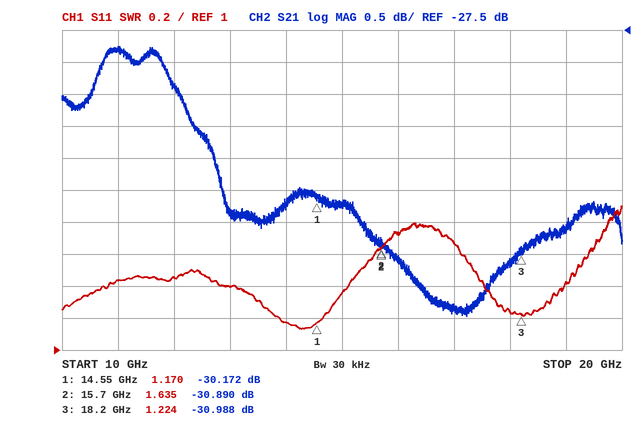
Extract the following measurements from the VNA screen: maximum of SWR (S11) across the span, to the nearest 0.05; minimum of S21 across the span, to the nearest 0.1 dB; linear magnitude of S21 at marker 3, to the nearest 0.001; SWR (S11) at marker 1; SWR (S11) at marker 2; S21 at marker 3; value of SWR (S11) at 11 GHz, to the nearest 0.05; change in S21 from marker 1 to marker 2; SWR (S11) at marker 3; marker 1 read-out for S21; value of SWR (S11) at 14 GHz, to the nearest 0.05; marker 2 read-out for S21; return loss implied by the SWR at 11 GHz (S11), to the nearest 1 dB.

1.90
-32.0 dB
0.028
1.170
1.635
-30.988 dB
1.45
-0.718 dB
1.224
-30.172 dB
1.15
-30.890 dB
15 dB
